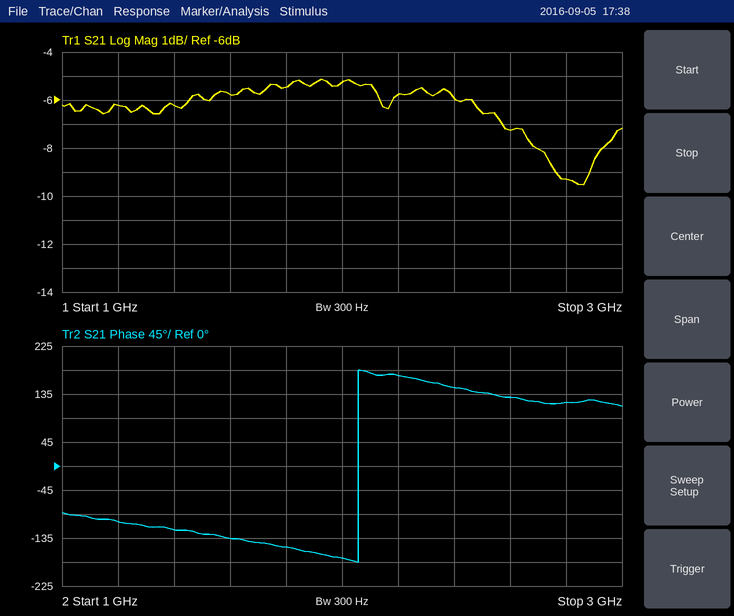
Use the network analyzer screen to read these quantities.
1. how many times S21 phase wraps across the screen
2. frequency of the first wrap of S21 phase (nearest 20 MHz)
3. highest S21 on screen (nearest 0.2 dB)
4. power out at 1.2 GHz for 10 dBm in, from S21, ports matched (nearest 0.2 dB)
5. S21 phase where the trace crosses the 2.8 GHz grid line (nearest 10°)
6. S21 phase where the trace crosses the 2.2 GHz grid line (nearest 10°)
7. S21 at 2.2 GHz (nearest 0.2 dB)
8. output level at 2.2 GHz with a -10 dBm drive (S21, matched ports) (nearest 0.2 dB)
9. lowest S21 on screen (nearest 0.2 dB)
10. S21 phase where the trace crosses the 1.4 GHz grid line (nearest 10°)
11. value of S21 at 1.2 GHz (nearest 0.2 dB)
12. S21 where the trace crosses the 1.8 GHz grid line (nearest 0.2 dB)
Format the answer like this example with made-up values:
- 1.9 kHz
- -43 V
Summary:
- 1
- 2.06 GHz
- -5.2 dB
- 3.8 dBm
- 120°
- 170°
- -5.8 dB
- -15.8 dBm
- -9.6 dB
- -120°
- -6.2 dB
- -5.4 dB
